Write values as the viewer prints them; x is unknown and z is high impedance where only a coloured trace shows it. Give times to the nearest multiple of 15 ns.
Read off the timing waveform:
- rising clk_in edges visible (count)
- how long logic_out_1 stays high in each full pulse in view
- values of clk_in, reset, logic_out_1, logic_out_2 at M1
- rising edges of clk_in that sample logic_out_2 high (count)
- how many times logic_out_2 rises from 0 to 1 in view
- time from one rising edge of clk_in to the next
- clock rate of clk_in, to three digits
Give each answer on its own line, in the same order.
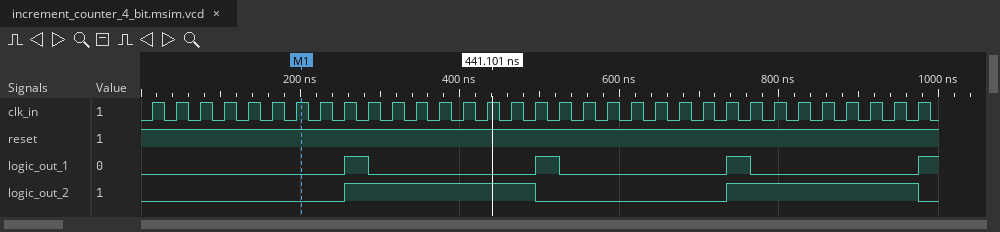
33
30 ns, 30 ns, 30 ns
clk_in=1, reset=1, logic_out_1=0, logic_out_2=0
16
2
30 ns
33.3 MHz
